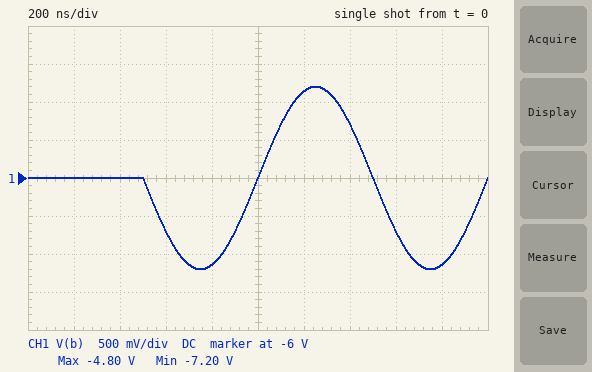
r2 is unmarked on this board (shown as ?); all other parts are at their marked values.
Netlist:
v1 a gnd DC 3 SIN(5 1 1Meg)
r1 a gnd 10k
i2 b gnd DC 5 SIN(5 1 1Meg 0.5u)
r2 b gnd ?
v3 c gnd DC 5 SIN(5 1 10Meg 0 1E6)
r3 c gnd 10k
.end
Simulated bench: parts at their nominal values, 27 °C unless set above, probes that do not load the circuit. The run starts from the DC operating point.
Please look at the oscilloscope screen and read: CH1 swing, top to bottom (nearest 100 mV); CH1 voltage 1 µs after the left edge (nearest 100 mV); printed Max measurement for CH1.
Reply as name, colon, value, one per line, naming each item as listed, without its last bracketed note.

CH1 swing, top to bottom: 2.4 V
CH1 voltage 1 µs after the left edge: -6.0 V
printed Max measurement for CH1: -4.80 V
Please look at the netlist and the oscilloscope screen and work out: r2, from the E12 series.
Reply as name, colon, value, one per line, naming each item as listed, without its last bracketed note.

r2, from the E12 series: 1.2 Ω
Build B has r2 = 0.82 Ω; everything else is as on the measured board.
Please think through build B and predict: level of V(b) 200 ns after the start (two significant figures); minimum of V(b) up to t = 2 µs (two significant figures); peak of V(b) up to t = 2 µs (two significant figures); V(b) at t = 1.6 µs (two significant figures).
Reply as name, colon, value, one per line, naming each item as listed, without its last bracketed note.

level of V(b) 200 ns after the start: -4.1 V
minimum of V(b) up to t = 2 µs: -4.9 V
peak of V(b) up to t = 2 µs: -3.3 V
V(b) at t = 1.6 µs: -4.6 V
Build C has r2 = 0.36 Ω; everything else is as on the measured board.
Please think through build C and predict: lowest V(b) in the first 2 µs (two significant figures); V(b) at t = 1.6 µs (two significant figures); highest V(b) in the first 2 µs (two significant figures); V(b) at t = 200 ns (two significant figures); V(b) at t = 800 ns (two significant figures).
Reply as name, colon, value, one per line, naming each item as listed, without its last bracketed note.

lowest V(b) in the first 2 µs: -2.2 V
V(b) at t = 1.6 µs: -2.0 V
highest V(b) in the first 2 µs: -1.4 V
V(b) at t = 200 ns: -1.8 V
V(b) at t = 800 ns: -2.1 V
